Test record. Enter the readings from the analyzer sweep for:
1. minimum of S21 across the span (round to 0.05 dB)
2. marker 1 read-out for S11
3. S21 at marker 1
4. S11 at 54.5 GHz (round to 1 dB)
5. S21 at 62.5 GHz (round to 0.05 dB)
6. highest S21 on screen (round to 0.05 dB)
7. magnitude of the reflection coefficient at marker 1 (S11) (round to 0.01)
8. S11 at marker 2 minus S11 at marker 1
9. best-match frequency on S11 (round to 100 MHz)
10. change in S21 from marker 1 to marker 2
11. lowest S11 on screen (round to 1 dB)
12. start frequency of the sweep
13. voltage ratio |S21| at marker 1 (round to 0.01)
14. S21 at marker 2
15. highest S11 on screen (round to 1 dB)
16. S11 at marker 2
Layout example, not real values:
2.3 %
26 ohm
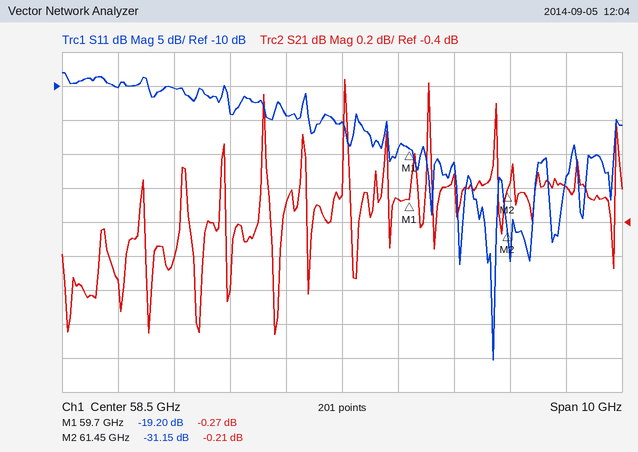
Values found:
-1.05 dB
-19.20 dB
-0.27 dB
-10 dB
-0.20 dB
0.45 dB
0.11
-11.95 dB
61.2 GHz
0.06 dB
-50 dB
53.5 GHz
0.97
-0.21 dB
-8 dB
-31.15 dB
